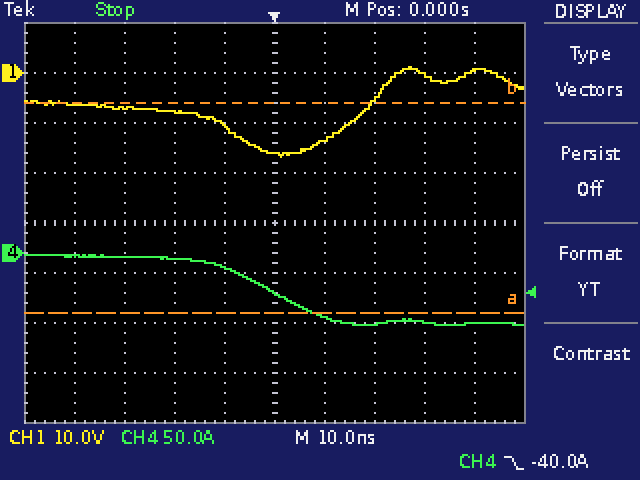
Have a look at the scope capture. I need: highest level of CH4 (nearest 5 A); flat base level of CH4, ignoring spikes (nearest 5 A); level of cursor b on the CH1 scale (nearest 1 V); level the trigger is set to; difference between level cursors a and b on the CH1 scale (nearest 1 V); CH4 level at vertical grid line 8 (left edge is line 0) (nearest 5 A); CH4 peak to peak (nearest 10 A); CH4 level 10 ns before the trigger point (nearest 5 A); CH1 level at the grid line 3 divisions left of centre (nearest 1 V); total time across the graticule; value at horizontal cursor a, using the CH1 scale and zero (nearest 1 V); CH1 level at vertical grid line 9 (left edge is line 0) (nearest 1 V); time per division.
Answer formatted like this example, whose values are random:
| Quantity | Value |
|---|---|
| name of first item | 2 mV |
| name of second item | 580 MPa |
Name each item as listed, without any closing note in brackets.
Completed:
| Quantity | Value |
|---|---|
| highest level of CH4 | 0 A |
| flat base level of CH4, ignoring spikes | -70 A |
| level of cursor b on the CH1 scale | -6 V |
| level the trigger is set to | -40.0 A |
| difference between level cursors a and b on the CH1 scale | 42 V |
| CH4 level at vertical grid line 8 (left edge is line 0) | -70 A |
| CH4 peak to peak | 70 A |
| CH4 level 10 ns before the trigger point | -15 A |
| CH1 level at the grid line 3 divisions left of centre | -7 V |
| total time across the graticule | 100 ns |
| value at horizontal cursor a, using the CH1 scale and zero | -48 V |
| CH1 level at vertical grid line 9 (left edge is line 0) | 0 V |
| time per division | 10 ns |
